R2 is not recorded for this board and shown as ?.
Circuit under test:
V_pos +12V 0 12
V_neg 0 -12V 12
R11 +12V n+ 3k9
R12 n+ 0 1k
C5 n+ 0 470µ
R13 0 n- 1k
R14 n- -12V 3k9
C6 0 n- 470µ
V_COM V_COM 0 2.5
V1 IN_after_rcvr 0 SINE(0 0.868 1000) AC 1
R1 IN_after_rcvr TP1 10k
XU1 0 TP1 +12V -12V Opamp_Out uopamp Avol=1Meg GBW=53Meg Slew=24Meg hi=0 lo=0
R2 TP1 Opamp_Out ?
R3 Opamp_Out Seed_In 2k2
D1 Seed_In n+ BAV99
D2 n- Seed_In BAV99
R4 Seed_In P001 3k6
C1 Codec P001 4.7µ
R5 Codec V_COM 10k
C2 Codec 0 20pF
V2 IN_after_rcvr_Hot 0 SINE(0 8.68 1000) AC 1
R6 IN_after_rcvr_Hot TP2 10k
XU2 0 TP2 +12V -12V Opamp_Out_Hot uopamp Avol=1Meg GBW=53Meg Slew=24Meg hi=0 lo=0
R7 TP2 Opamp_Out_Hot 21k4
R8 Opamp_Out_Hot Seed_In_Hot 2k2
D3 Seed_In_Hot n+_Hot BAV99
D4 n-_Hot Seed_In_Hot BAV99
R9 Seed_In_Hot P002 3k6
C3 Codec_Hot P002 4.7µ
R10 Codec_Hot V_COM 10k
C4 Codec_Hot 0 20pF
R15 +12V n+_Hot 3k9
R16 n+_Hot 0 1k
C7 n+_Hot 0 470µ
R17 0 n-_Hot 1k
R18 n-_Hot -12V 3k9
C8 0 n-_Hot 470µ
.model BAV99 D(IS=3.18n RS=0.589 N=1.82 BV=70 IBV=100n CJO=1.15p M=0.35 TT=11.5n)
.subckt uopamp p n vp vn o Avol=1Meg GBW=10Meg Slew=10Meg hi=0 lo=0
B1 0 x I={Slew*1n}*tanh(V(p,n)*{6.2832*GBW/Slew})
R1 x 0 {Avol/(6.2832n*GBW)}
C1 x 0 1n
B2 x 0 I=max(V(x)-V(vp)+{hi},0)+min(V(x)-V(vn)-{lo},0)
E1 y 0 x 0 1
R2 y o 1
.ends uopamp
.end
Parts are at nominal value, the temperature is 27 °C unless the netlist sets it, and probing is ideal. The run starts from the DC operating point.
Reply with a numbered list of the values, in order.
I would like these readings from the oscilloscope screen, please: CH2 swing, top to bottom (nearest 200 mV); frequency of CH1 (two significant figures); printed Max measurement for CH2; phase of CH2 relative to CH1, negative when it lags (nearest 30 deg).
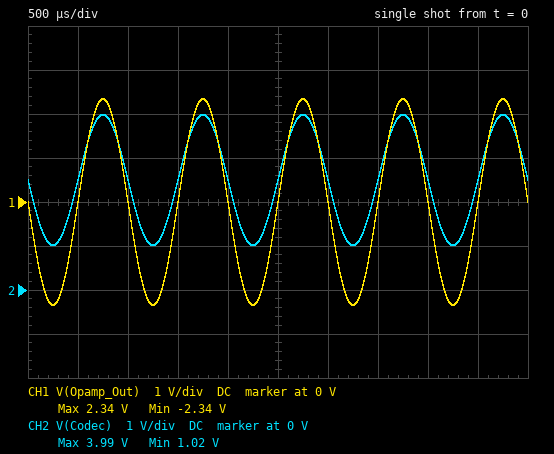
1. 3.0 V
2. 1.0 kHz
3. 3.99 V
4. 0 deg
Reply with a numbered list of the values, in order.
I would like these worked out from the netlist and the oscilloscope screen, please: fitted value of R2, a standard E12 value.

1. 27 kΩ
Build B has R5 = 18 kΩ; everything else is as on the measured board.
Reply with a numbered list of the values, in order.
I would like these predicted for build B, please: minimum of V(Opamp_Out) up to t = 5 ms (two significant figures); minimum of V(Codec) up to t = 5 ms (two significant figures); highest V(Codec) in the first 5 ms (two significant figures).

1. -2.3 V
2. 730 mV
3. 4.3 V
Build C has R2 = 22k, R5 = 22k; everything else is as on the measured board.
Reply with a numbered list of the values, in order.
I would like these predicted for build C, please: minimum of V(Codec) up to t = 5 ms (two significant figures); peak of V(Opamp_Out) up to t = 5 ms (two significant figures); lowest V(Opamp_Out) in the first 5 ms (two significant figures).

1. 990 mV
2. 1.9 V
3. -1.9 V
